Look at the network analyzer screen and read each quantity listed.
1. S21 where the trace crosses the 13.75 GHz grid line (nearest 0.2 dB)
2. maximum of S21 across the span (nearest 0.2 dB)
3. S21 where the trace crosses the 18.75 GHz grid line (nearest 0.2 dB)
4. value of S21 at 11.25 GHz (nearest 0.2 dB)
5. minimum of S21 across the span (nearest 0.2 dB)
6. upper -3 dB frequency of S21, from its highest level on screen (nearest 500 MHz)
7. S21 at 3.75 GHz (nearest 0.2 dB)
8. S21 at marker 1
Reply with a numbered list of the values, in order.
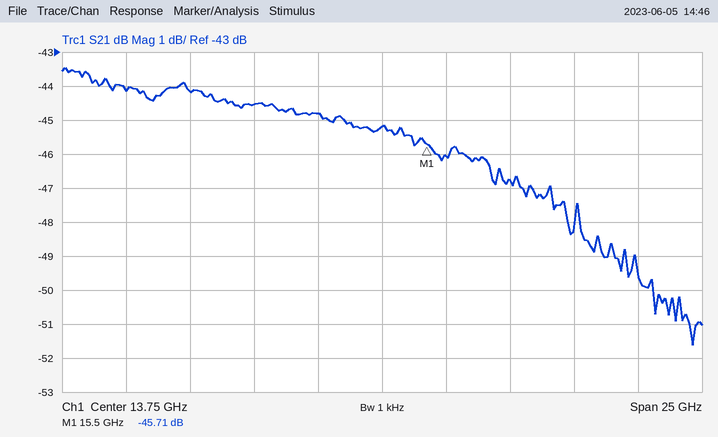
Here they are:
1. -45.2 dB
2. -43.4 dB
3. -46.8 dB
4. -44.8 dB
5. -51.6 dB
6. 18.0 GHz
7. -44.2 dB
8. -45.71 dB
